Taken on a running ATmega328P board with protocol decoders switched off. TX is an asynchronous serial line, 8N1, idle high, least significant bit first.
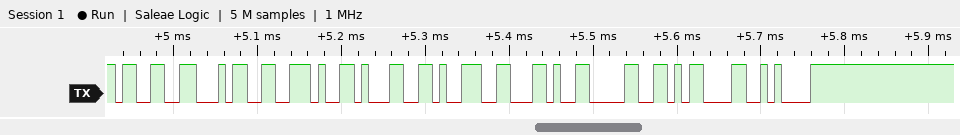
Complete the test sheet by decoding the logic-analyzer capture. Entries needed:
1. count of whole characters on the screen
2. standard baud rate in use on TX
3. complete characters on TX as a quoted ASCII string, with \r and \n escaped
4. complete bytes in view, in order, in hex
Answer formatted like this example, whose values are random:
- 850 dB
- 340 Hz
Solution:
- 9
- 115200 baud
- "34.19,0\r\n"
- 33 34 2E 31 39 2C 30 0D 0A
